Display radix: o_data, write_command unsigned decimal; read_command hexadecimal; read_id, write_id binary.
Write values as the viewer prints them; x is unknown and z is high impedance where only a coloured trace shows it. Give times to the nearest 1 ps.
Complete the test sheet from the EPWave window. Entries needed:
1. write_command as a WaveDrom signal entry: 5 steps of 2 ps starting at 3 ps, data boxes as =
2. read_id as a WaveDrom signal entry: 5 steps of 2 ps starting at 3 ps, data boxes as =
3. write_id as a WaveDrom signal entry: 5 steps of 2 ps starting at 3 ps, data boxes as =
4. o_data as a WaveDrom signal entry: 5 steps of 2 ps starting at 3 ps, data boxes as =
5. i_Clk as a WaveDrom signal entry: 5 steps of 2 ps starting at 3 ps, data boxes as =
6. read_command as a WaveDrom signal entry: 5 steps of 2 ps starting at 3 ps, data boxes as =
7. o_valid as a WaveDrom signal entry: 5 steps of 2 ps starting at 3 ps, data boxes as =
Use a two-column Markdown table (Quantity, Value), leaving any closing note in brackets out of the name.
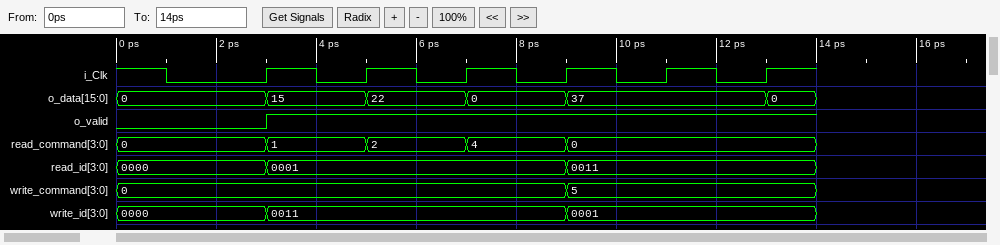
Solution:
| Quantity | Value |
|---|---|
| write_command as a WaveDrom signal entry: 5 steps of 2 ps starting at 3 ps, data boxes as = | {name: 'write_command', wave: '=..=.', data: '0 5'} |
| read_id as a WaveDrom signal entry: 5 steps of 2 ps starting at 3 ps, data boxes as = | {name: 'read_id', wave: '=..=.', data: '0001 0011'} |
| write_id as a WaveDrom signal entry: 5 steps of 2 ps starting at 3 ps, data boxes as = | {name: 'write_id', wave: '=..=.', data: '0011 0001'} |
| o_data as a WaveDrom signal entry: 5 steps of 2 ps starting at 3 ps, data boxes as = | {name: 'o_data', wave: '====.', data: '15 22 0 37'} |
| i_Clk as a WaveDrom signal entry: 5 steps of 2 ps starting at 3 ps, data boxes as = | {name: 'i_Clk', wave: 'p....'} |
| read_command as a WaveDrom signal entry: 5 steps of 2 ps starting at 3 ps, data boxes as = | {name: 'read_command', wave: '====.', data: '1 2 4 0'} |
| o_valid as a WaveDrom signal entry: 5 steps of 2 ps starting at 3 ps, data boxes as = | {name: 'o_valid', wave: '1....'} |
